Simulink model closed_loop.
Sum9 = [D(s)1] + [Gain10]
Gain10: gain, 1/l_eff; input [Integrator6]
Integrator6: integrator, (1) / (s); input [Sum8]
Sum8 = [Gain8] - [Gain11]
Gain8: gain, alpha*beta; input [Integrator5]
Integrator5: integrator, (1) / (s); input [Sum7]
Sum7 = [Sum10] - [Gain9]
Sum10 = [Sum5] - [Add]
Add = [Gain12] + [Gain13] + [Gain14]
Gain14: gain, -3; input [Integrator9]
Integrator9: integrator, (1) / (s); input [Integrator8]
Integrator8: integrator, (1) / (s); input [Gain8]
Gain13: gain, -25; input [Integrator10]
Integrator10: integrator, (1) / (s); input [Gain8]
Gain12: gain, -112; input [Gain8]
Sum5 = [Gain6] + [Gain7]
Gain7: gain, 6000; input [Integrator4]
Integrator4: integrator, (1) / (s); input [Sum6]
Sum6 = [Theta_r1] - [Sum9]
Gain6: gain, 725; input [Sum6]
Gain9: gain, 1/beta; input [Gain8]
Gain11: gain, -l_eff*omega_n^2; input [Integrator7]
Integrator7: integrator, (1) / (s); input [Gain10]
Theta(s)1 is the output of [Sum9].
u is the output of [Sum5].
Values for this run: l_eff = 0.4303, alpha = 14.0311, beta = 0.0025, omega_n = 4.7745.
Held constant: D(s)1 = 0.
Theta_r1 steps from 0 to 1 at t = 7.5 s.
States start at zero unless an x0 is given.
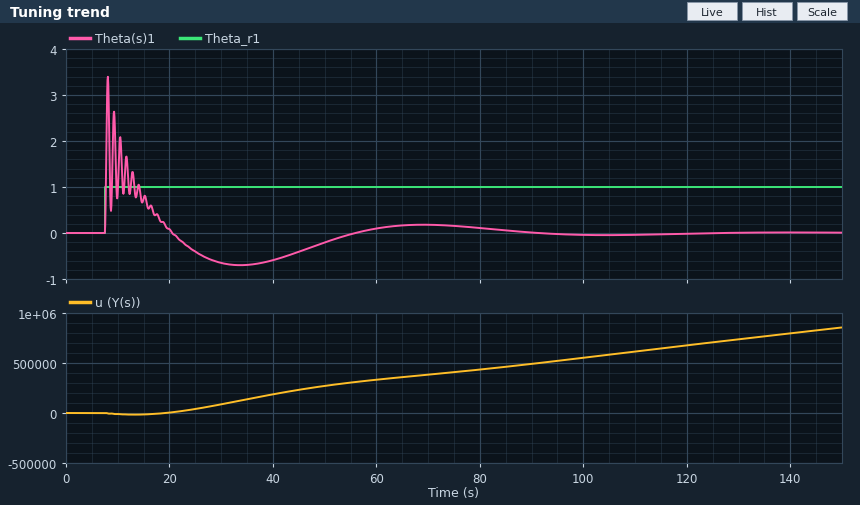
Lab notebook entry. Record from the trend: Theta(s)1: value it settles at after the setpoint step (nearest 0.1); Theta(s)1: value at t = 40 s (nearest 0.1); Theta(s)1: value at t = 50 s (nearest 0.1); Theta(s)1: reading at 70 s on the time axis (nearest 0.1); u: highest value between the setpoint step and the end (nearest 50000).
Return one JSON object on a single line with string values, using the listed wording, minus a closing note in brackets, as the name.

{"Theta(s)1: value it settles at after the setpoint step": "0.0", "Theta(s)1: value at t = 40 s": "-0.6", "Theta(s)1: value at t = 50 s": "-0.2", "Theta(s)1: reading at 70 s on the time axis": "0.2", "u: highest value between the setpoint step and the end": "850000"}
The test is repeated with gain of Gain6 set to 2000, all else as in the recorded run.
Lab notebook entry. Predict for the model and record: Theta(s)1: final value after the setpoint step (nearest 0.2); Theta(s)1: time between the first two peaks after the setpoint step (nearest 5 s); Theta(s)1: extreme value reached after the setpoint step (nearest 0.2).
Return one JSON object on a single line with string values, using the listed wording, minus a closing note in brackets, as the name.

{"Theta(s)1: final value after the setpoint step": "0.0", "Theta(s)1: time between the first two peaks after the setpoint step": "60 s", "Theta(s)1: extreme value reached after the setpoint step": "2.0"}
